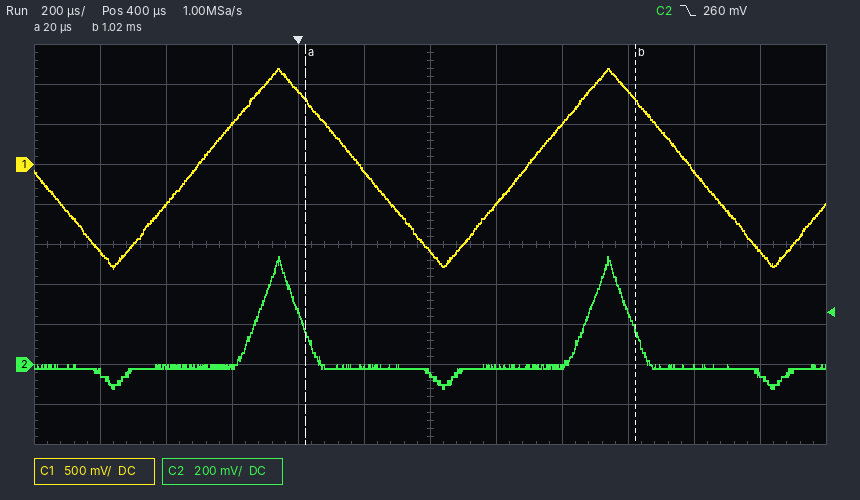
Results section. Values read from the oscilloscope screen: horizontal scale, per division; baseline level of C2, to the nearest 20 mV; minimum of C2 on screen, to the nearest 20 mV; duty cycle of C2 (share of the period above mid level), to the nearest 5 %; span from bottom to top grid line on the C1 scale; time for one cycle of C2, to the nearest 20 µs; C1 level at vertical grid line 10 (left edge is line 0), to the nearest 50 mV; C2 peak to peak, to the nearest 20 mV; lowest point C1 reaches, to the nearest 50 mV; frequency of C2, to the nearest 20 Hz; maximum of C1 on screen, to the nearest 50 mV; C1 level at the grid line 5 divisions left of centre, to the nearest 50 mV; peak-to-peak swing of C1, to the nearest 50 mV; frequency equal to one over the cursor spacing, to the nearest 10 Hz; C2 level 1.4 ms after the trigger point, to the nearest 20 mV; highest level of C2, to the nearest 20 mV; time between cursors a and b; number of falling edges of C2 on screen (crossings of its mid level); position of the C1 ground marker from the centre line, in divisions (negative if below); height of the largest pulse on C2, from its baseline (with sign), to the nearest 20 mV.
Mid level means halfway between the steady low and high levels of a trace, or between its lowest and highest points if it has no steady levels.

200 µs
-20 mV
-120 mV
15 %
5 V
1.00 ms
-100 mV
660 mV
-1.30 V
1.00 kHz
1.20 V
-1.10 V
2.50 V
1.00 kHz
-40 mV
540 mV
1.00 ms
2
+2.0 div
+560 mV
